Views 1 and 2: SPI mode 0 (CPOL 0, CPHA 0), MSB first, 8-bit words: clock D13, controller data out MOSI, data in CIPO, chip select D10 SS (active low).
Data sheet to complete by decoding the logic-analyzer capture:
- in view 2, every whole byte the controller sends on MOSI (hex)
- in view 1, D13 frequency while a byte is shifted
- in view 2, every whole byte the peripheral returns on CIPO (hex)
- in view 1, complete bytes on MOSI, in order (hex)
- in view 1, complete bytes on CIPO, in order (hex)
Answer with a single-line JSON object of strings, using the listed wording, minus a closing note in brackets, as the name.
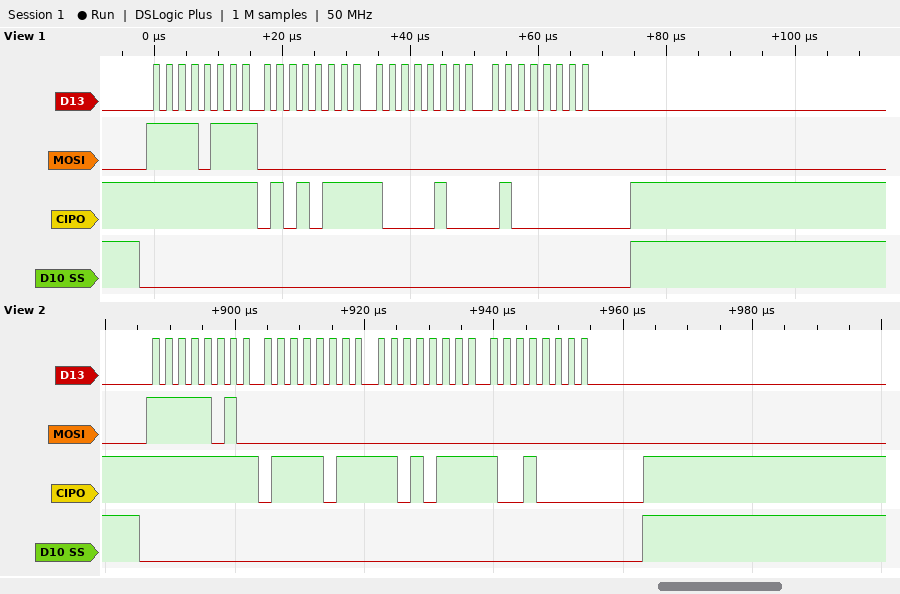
{"in view 2, every whole byte the controller sends on MOSI": "0xFA 0x00 0x00 0x00", "in view 1, D13 frequency while a byte is shifted": "500 kHz", "in view 2, every whole byte the peripheral returns on CIPO": "0xFF 0x7B 0xD7 0x90", "in view 1, complete bytes on MOSI, in order": "F7 00 00 00", "in view 1, complete bytes on CIPO, in order": "FF 57 84 40"}
